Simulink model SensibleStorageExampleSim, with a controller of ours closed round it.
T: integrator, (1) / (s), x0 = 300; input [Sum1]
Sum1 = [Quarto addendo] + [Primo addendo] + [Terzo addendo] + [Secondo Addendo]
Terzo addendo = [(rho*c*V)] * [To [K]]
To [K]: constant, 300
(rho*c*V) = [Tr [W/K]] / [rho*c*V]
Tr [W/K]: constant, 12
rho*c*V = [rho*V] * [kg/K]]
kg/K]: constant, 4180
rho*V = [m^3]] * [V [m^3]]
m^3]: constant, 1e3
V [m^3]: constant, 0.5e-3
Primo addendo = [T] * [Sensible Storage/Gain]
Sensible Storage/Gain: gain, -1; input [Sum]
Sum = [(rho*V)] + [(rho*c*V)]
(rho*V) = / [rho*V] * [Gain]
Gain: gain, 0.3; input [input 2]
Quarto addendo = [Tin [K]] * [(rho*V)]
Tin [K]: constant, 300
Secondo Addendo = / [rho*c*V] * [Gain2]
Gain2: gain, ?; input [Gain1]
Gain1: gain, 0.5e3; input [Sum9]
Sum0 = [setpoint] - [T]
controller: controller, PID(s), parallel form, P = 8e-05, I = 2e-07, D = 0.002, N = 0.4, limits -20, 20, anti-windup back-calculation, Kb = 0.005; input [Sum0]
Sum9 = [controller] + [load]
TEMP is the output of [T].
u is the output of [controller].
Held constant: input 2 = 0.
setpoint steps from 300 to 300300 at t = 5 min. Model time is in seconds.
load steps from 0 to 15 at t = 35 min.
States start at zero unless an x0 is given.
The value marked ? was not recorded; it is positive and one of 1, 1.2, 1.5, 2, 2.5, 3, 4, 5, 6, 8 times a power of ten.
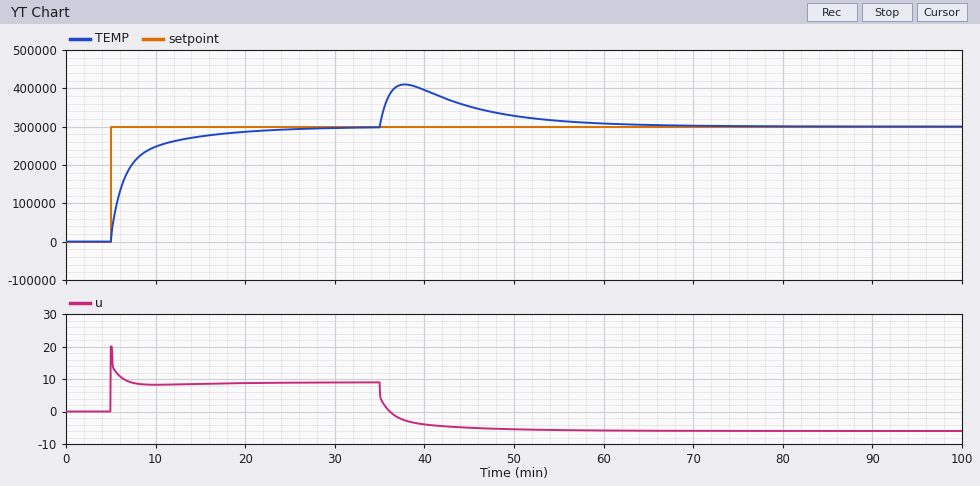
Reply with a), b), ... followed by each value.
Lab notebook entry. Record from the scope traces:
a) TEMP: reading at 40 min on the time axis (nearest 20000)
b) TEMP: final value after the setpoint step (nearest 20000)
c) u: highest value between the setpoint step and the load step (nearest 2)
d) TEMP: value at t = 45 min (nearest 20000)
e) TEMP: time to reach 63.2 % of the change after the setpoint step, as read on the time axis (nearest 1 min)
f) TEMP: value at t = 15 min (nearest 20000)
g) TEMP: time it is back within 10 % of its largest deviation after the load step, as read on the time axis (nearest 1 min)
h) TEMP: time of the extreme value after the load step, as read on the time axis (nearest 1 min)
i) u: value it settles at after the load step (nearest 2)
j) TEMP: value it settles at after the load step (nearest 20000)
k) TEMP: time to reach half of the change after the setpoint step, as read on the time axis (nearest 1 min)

a) 400000
b) 300000
c) 20
d) 360000
e) 7 min
f) 280000
g) 57 min
h) 38 min
i) -6
j) 300000
k) 6 min
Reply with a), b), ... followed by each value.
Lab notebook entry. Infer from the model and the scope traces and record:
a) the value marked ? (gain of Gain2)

a) 800
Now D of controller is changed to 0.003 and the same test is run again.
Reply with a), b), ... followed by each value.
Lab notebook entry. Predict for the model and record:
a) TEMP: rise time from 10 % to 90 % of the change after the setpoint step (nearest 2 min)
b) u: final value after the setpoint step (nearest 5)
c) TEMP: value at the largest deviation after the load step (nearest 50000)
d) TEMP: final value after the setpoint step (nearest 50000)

a) 10 min
b) 10
c) 400000
d) 300000
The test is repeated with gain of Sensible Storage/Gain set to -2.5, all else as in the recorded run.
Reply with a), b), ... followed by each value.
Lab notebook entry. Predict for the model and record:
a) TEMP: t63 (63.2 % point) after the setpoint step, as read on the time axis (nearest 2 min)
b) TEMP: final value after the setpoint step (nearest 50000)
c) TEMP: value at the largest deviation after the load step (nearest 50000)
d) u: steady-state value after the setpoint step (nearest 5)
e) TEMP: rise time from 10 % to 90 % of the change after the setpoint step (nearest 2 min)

a) 8 min
b) 250000
c) 350000
d) 20
e) 12 min
